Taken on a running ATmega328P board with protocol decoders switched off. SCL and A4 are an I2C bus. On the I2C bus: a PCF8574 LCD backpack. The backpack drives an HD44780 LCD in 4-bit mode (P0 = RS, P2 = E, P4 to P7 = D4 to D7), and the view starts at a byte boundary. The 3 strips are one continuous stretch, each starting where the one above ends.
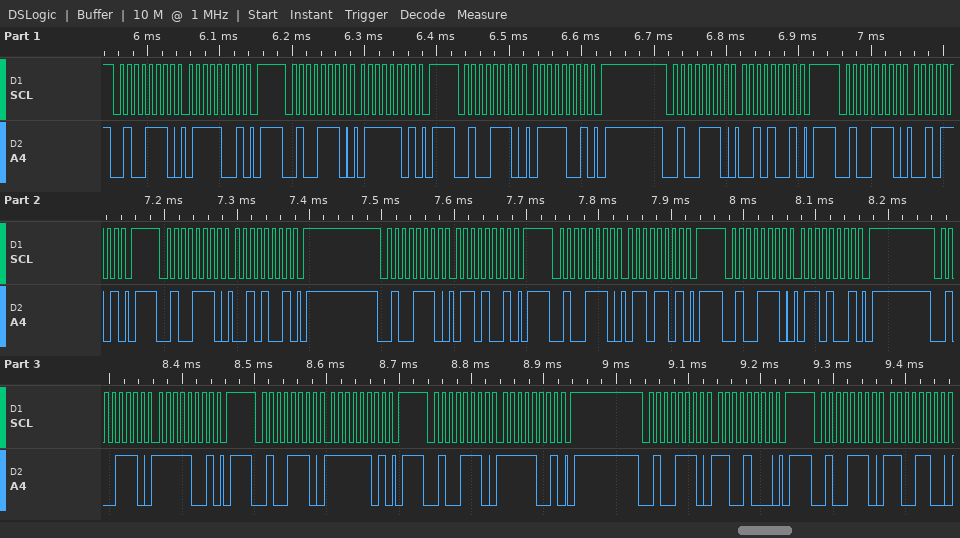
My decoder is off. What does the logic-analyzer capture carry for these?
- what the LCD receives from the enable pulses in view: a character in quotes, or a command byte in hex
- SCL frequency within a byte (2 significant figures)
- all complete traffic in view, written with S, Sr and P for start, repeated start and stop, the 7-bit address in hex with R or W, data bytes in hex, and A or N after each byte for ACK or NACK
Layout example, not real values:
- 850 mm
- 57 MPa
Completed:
- 'r' 'o'
- 100 kHz
- S 27W A 79 A P S 27W A 7D A P S 27W A 79 A P S 27W A 29 A P S 27W A 2D A P S 27W A 29 A P S 27W A 69 A P S 27W A 6D A P S 27W A 69 A P S 27W A F9 A P S 27W A FD A P S 27W A F9 A P S 27W A C8 A P S 27W A CC A
